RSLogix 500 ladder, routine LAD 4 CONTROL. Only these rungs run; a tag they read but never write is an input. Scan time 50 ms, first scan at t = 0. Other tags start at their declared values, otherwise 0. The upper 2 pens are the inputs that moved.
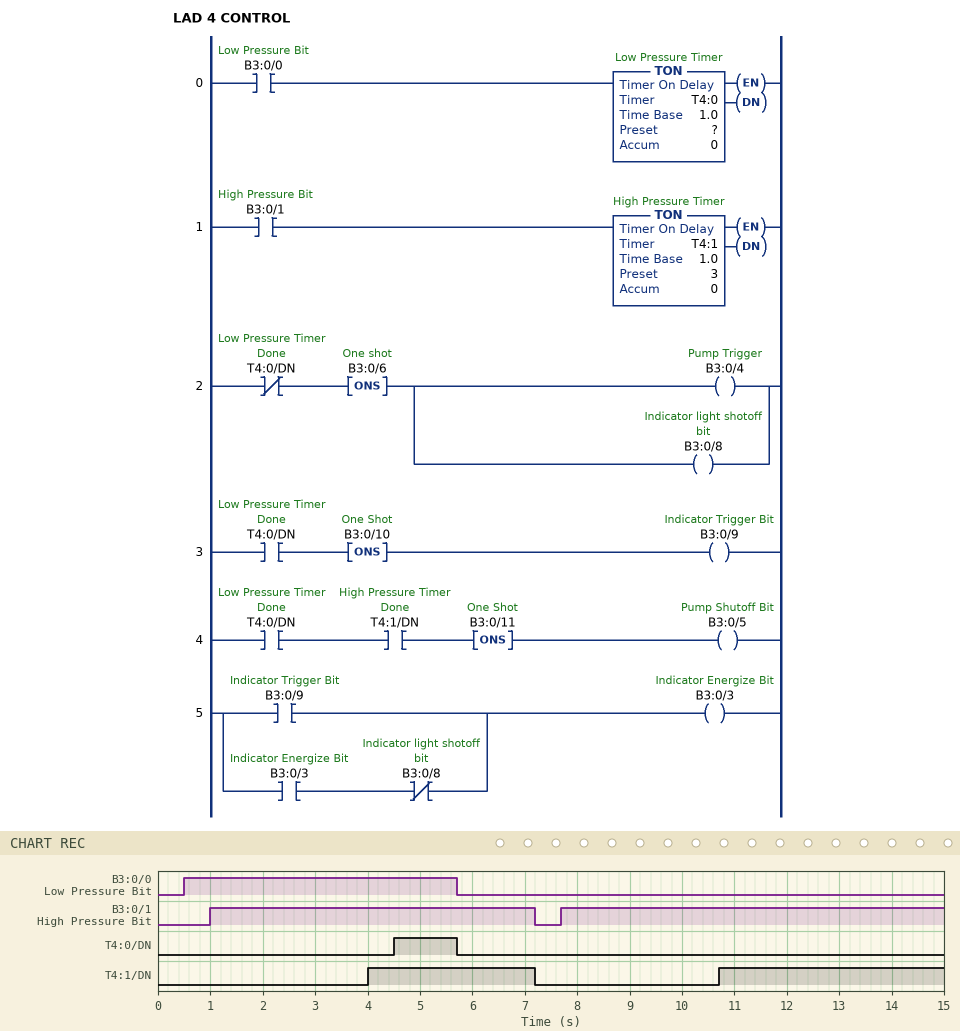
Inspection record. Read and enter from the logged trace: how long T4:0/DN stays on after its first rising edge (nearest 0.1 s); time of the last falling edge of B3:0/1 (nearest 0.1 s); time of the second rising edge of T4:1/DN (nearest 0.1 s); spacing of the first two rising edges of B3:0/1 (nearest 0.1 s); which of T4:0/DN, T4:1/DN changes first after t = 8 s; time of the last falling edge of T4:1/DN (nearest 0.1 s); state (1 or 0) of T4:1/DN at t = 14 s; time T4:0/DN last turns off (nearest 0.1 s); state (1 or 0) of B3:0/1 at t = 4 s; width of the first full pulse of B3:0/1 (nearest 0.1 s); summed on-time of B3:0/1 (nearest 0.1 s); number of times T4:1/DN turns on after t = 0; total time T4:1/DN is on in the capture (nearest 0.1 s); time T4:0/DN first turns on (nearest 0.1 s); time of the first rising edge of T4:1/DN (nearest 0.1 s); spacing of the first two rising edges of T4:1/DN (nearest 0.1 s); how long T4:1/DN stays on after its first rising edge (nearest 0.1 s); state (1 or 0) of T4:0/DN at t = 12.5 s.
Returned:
1.2 s
7.2 s
10.7 s
6.7 s
T4:1/DN
7.2 s
1
5.7 s
1
6.2 s
13.5 s
2
7.5 s
4.5 s
4.0 s
6.7 s
3.2 s
0
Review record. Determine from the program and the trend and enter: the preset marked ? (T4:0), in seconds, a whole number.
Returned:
4 s
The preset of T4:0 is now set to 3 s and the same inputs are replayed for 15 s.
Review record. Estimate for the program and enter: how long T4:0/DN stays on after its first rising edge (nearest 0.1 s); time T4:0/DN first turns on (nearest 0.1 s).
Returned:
2.2 s
3.5 s
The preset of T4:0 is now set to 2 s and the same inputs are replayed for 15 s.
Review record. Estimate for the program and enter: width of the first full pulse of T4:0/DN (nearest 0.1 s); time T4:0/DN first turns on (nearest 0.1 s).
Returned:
3.2 s
2.5 s
